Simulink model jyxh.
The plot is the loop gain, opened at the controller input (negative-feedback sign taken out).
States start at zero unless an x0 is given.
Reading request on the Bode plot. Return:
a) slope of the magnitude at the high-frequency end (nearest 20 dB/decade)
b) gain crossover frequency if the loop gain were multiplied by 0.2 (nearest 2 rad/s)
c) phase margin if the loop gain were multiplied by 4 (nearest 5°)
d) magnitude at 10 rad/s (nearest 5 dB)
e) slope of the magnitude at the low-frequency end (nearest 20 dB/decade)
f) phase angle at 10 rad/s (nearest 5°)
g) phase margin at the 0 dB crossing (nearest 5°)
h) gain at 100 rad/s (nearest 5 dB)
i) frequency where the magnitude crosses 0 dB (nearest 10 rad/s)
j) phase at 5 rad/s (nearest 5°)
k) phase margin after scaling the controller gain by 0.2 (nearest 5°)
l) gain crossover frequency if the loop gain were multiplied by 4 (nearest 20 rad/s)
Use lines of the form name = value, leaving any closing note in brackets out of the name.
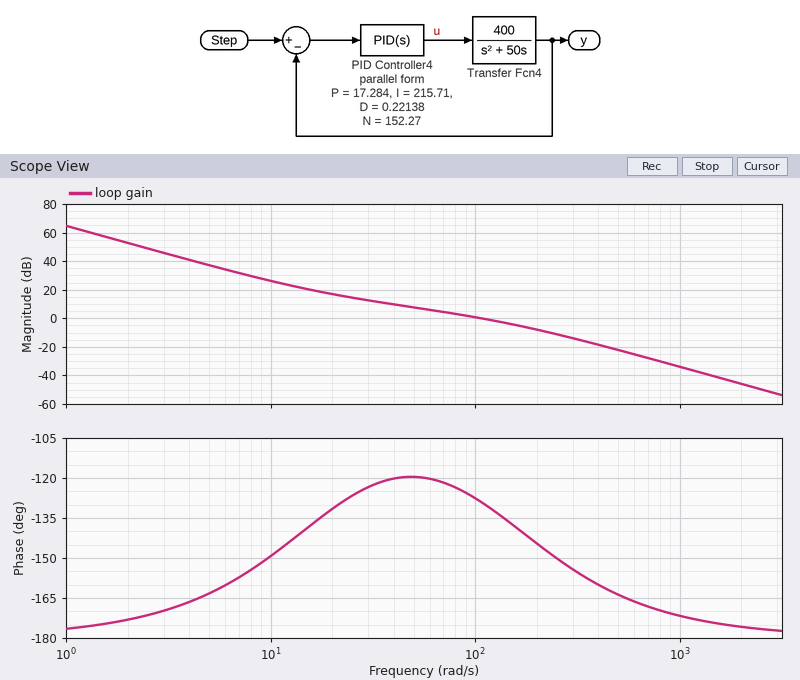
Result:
slope of the magnitude at the high-frequency end = -40 dB/decade
gain crossover frequency if the loop gain were multiplied by 0.2 = 26 rad/s
phase margin if the loop gain were multiplied by 4 = 30°
magnitude at 10 rad/s = 25 dB
slope of the magnitude at the low-frequency end = -40 dB/decade
phase angle at 10 rad/s = -150°
phase margin at the 0 dB crossing = 50°
gain at 100 rad/s = 0 dB
frequency where the magnitude crosses 0 dB = 110 rad/s
phase at 5 rad/s = -165°
phase margin after scaling the controller gain by 0.2 = 55°
gain crossover frequency if the loop gain were multiplied by 4 = 260 rad/s
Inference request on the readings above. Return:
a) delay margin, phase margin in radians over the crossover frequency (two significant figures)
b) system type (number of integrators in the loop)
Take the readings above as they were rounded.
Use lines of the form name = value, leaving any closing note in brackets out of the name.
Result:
delay margin, phase margin in radians over the crossover frequency = 0.0079 s
system type = 2
